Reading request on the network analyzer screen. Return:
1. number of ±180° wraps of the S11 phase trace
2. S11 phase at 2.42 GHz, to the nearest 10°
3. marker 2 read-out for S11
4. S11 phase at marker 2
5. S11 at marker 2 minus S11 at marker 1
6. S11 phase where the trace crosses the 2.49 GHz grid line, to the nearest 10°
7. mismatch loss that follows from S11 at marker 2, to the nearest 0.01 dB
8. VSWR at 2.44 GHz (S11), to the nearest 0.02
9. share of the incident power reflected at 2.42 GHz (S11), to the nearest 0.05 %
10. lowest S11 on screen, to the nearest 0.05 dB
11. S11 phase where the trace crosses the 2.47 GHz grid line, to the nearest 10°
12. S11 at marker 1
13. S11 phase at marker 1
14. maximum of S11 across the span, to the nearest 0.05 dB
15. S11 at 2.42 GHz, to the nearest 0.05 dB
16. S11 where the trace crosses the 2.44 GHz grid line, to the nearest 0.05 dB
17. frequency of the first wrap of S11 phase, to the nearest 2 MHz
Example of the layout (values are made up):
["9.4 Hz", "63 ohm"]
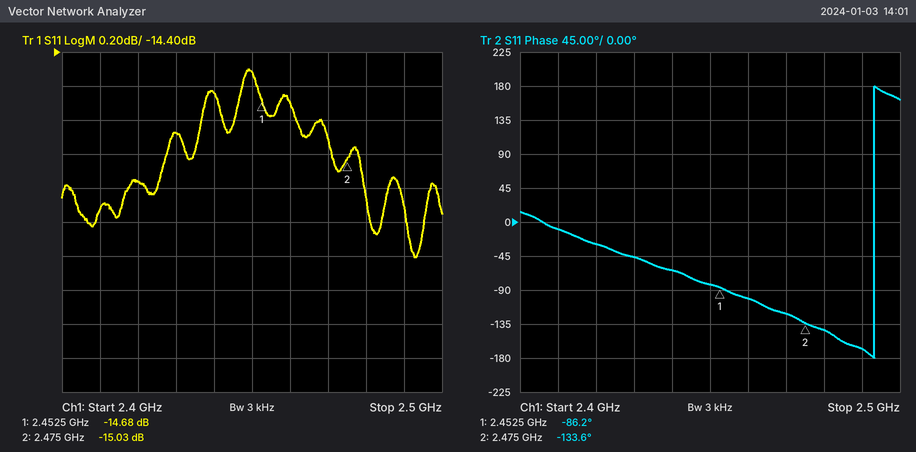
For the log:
["1", "-30°", "-15.03 dB", "-133.6°", "-0.35 dB", "-170°", "0.14 dB", "1.46", "3.05 %", "-15.60 dB", "-120°", "-14.68 dB", "-86.2°", "-14.50 dB", "-15.15 dB", "-14.65 dB", "2.494 GHz"]
